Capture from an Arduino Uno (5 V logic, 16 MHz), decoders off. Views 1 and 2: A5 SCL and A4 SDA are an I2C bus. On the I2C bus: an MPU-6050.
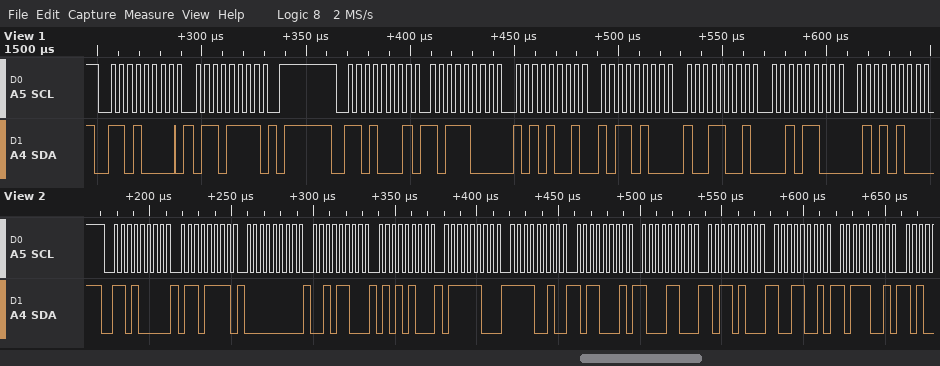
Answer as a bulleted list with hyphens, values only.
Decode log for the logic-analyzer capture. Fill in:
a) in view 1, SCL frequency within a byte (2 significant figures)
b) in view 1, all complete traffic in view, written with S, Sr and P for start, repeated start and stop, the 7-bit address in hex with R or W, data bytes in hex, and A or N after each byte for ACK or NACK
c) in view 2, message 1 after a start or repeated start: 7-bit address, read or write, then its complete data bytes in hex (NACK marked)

- 250 kHz
- S 68W A 6F A P S 68R A B8 A A9 A B4 A 99 A 2C A 54 A
- 0x68 write: 6F 00 2C 54 7C F2 B1 8C B4 99 B9
